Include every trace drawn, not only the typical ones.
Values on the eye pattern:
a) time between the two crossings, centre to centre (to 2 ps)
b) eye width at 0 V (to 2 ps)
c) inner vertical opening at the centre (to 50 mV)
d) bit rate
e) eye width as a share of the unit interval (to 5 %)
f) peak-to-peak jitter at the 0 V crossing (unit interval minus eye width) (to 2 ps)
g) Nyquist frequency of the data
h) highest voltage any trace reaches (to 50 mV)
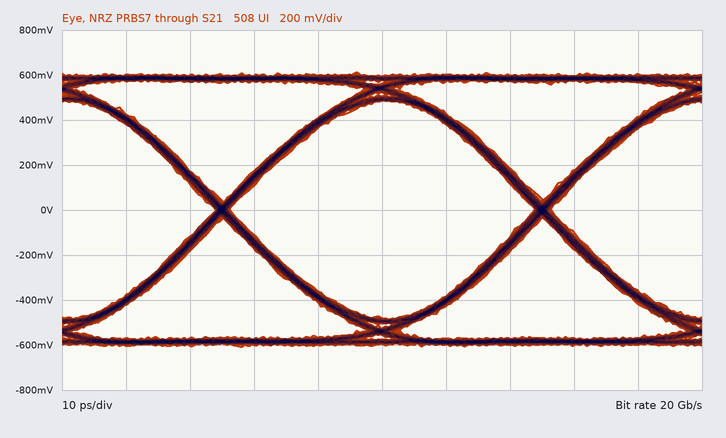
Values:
50 ps
48 ps
950 mV
20 Gb/s
95 %
2 ps
10 GHz
600 mV
